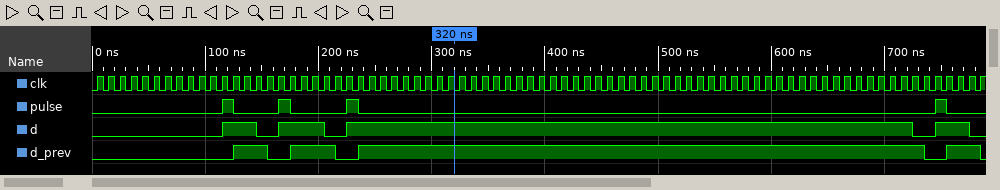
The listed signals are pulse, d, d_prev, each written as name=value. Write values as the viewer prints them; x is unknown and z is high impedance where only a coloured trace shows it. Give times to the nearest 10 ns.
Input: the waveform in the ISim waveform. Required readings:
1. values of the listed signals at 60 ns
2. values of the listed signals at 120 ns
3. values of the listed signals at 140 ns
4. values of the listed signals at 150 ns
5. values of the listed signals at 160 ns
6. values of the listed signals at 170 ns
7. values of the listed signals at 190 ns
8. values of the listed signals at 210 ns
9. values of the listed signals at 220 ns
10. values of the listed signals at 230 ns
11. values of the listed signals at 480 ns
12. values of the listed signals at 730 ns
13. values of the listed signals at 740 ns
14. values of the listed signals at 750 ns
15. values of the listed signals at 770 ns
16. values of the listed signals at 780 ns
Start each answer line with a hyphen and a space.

- pulse=0, d=0, d_prev=0
- pulse=1, d=1, d_prev=0
- pulse=0, d=1, d_prev=1
- pulse=0, d=0, d_prev=1
- pulse=0, d=0, d_prev=0
- pulse=1, d=1, d_prev=0
- pulse=0, d=1, d_prev=1
- pulse=0, d=0, d_prev=1
- pulse=0, d=0, d_prev=0
- pulse=1, d=1, d_prev=0
- pulse=0, d=1, d_prev=1
- pulse=0, d=0, d_prev=1
- pulse=0, d=0, d_prev=0
- pulse=1, d=1, d_prev=0
- pulse=0, d=1, d_prev=1
- pulse=0, d=0, d_prev=1
